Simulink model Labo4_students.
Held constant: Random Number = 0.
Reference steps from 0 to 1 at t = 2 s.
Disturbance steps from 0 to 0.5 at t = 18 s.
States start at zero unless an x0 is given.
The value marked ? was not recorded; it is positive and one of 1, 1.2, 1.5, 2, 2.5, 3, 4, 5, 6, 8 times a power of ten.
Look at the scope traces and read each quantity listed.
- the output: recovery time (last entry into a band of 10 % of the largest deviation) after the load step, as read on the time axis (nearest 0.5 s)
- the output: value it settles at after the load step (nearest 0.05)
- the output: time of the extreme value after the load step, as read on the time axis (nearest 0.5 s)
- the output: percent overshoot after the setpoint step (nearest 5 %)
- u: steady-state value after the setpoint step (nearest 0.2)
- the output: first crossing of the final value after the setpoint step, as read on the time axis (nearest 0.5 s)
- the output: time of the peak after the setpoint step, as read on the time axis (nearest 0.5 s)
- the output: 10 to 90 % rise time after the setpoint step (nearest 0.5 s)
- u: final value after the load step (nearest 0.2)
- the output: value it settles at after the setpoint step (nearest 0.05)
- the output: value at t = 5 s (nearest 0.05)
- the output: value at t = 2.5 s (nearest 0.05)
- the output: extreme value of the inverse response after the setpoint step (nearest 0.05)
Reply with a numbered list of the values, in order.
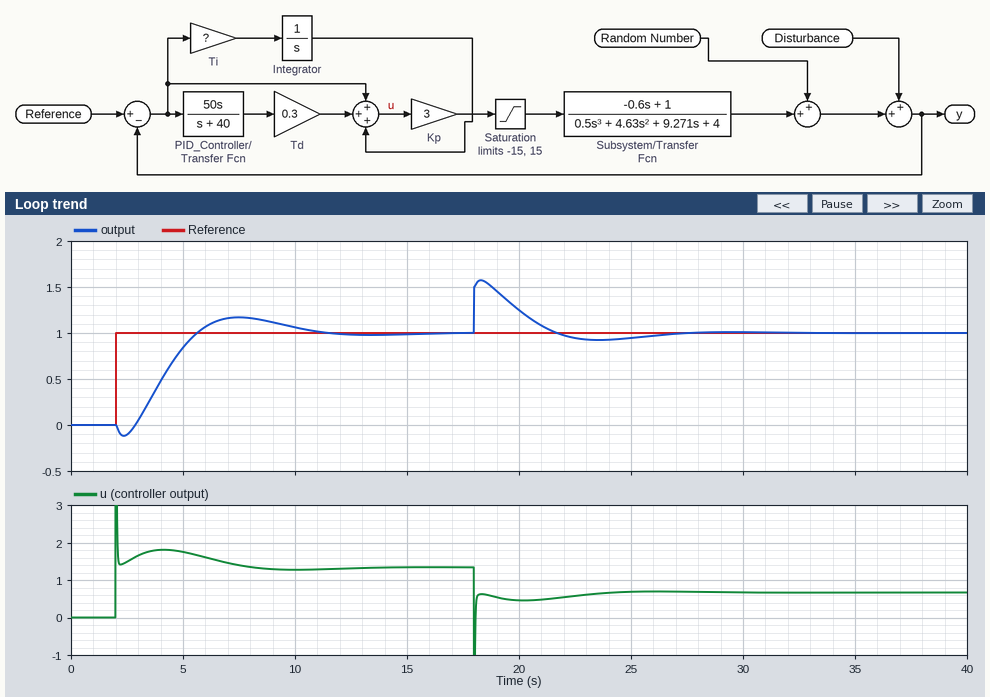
1. 25.0 s
2. 1.00
3. 18.5 s
4. 15 %
5. 1.4
6. 5.5 s
7. 7.5 s
8. 2.0 s
9. 0.6
10. 1.00
11. 0.85
12. -0.10
13. -0.10
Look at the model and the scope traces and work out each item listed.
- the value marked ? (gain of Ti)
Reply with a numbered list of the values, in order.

1. 0.8
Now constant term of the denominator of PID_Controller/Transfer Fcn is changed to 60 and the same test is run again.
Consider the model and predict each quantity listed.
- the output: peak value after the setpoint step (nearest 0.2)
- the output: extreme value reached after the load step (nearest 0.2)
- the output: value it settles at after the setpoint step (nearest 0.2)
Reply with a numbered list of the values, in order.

1. 1.2
2. 1.6
3. 1.0
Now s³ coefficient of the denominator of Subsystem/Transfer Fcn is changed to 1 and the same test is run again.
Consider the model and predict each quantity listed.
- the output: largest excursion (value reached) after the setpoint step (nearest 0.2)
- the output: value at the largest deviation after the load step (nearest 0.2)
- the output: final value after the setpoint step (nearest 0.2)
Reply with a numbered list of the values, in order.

1. 1.2
2. 1.6
3. 1.0
